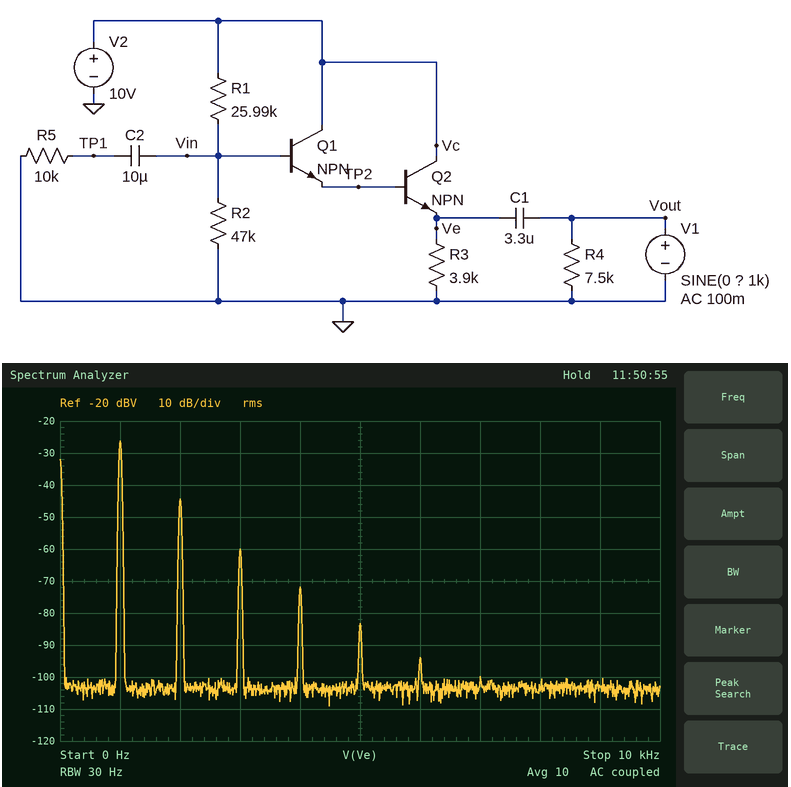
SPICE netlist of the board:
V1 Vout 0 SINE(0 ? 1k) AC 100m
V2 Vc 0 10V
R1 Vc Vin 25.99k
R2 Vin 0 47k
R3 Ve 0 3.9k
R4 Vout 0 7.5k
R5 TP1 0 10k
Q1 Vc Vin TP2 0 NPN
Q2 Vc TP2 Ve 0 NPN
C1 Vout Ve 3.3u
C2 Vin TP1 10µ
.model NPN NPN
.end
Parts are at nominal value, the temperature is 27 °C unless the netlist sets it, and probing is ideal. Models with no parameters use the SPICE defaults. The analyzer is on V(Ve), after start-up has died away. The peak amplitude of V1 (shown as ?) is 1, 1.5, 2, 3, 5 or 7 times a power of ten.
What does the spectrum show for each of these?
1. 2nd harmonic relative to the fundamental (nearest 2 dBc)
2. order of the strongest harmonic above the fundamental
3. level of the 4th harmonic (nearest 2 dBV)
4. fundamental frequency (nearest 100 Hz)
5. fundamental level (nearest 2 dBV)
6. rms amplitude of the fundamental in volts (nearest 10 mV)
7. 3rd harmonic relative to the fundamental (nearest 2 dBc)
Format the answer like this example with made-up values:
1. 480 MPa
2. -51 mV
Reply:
1. -18 dBc
2. 2
3. -72 dBV
4. 1.0 kHz
5. -26 dBV
6. 50 mV
7. -34 dBc
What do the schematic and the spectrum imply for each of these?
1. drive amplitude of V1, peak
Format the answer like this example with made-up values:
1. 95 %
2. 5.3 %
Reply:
1. 100 mV
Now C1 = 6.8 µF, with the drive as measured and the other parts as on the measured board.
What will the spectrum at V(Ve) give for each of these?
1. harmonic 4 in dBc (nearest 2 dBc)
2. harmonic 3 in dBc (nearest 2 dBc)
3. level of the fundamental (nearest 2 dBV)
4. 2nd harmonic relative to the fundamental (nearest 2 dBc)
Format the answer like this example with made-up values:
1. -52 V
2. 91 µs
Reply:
1. -50 dBc
2. -38 dBc
3. -24 dBV
4. -22 dBc
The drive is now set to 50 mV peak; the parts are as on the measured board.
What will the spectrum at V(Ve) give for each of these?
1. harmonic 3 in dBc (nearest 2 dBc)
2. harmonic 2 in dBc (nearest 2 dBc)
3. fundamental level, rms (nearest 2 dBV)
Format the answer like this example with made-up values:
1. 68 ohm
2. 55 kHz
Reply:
1. -44 dBc
2. -22 dBc
3. -32 dBV
